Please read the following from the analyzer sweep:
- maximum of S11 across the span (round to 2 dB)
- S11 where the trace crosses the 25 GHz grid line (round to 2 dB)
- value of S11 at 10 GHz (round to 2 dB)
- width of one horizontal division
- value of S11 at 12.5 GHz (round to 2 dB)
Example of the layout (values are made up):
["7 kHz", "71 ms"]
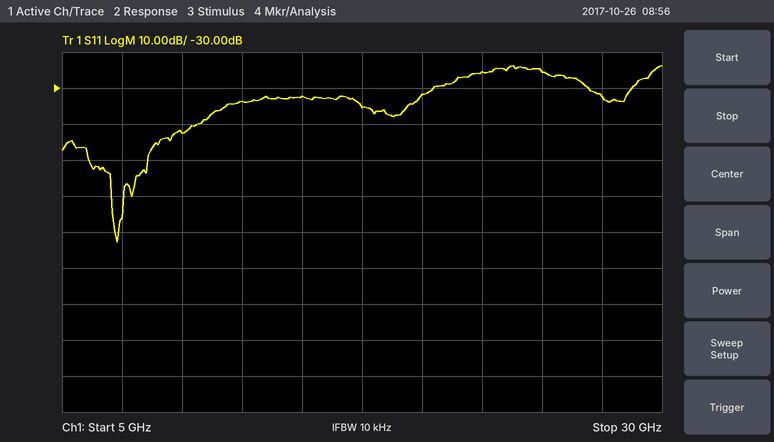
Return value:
["-24 dB", "-26 dB", "-42 dB", "2.5 GHz", "-34 dB"]
